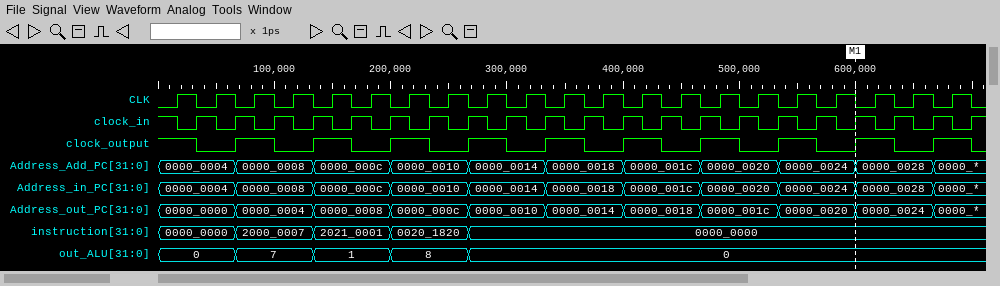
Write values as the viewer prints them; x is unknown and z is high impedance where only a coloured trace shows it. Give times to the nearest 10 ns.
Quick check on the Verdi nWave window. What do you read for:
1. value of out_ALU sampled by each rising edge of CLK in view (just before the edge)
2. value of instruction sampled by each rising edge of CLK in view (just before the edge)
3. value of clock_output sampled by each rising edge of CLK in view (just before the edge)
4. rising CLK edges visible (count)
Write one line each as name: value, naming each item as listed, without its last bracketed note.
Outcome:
value of out_ALU sampled by each rising edge of CLK in view: 0, 0, 7, 7, 1, 1, 8, 8, 0, 0, 0, 0, 0, 0, 0, 0, 0, 0, 0, 0, 0
value of instruction sampled by each rising edge of CLK in view: 0000_0000, 0000_0000, 2000_0007, 2000_0007, 2021_0001, 2021_0001, 0020_1820, 0020_1820, 0000_0000, 0000_0000, 0000_0000, 0000_0000, 0000_0000, 0000_0000, 0000_0000, 0000_0000, 0000_0000, 0000_0000, 0000_0000, 0000_0000, 0000_0000
value of clock_output sampled by each rising edge of CLK in view: 1 0 1 0 1 0 1 0 1 0 1 0 1 0 1 0 1 0 1 0 1
rising CLK edges visible: 21
